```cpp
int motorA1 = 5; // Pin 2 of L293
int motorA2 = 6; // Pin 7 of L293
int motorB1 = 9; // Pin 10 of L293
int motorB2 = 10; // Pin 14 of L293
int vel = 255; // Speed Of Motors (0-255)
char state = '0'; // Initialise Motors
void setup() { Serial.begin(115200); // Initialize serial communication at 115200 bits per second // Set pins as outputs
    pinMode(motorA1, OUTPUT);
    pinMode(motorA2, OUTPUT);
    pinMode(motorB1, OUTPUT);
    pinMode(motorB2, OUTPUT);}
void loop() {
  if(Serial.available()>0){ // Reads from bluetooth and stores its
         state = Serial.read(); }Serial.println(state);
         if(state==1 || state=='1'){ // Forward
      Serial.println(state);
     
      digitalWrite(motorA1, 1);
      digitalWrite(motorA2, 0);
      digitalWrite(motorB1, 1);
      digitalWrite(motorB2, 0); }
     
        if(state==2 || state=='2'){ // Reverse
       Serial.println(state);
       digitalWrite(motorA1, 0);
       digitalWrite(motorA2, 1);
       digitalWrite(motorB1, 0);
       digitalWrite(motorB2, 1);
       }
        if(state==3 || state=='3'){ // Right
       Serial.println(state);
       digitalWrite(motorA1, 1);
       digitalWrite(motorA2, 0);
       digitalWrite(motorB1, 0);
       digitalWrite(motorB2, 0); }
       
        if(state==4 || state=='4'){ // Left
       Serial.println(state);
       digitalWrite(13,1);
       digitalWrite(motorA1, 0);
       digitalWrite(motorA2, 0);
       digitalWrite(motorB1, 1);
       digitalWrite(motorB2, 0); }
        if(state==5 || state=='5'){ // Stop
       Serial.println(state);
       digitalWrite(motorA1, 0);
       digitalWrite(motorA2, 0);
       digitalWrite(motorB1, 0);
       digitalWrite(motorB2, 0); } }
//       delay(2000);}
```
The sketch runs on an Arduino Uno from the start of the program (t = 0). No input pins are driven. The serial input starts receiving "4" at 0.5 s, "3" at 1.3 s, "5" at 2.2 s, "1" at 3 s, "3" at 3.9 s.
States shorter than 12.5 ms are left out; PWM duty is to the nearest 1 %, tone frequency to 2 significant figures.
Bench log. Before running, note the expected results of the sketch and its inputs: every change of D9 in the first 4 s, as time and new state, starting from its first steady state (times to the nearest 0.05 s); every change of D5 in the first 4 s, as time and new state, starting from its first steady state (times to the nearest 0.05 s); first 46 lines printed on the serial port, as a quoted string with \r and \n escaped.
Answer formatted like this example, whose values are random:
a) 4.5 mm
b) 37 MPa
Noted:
a) 0 s low; 0.5 s high; 1.3 s low; 3 s high; 3.9 s low
b) 0 s low; 1.3 s high; 2.2 s low; 3 s high
c) "0\r\n0\r\n0\r\n0\r\n0\r\n0\r\n0\r\n0\r\n0\r\n0\r\n0\r\n0\r\n0\r\n0\r\n0\r\n0\r\n0\r\n0\r\n0\r\n0\r\n0\r\n0\r\n0\r\n0\r\n0\r\n0\r\n0\r\n0\r\n0\r\n0\r\n0\r\n0\r\n0\r\n0\r\n0\r\n0\r\n0\r\n0\r\n0\r\n0\r\n0\r\n0\r\n0\r\n0\r\n0\r\n0\r\n"
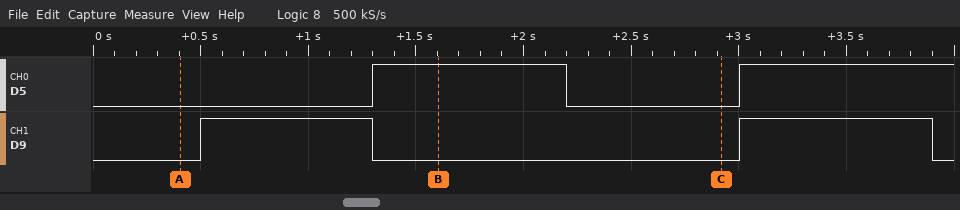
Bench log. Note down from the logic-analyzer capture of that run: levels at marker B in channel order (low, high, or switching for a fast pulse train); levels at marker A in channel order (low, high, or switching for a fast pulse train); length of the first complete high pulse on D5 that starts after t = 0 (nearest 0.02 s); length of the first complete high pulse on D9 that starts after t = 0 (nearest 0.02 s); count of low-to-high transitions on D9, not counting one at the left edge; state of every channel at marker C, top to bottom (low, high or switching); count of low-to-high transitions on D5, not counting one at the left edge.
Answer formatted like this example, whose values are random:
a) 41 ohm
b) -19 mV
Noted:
a) D5 high, D9 low
b) D5 low, D9 low
c) 0.90 s
d) 0.80 s
e) 2
f) D5 low, D9 low
g) 2
